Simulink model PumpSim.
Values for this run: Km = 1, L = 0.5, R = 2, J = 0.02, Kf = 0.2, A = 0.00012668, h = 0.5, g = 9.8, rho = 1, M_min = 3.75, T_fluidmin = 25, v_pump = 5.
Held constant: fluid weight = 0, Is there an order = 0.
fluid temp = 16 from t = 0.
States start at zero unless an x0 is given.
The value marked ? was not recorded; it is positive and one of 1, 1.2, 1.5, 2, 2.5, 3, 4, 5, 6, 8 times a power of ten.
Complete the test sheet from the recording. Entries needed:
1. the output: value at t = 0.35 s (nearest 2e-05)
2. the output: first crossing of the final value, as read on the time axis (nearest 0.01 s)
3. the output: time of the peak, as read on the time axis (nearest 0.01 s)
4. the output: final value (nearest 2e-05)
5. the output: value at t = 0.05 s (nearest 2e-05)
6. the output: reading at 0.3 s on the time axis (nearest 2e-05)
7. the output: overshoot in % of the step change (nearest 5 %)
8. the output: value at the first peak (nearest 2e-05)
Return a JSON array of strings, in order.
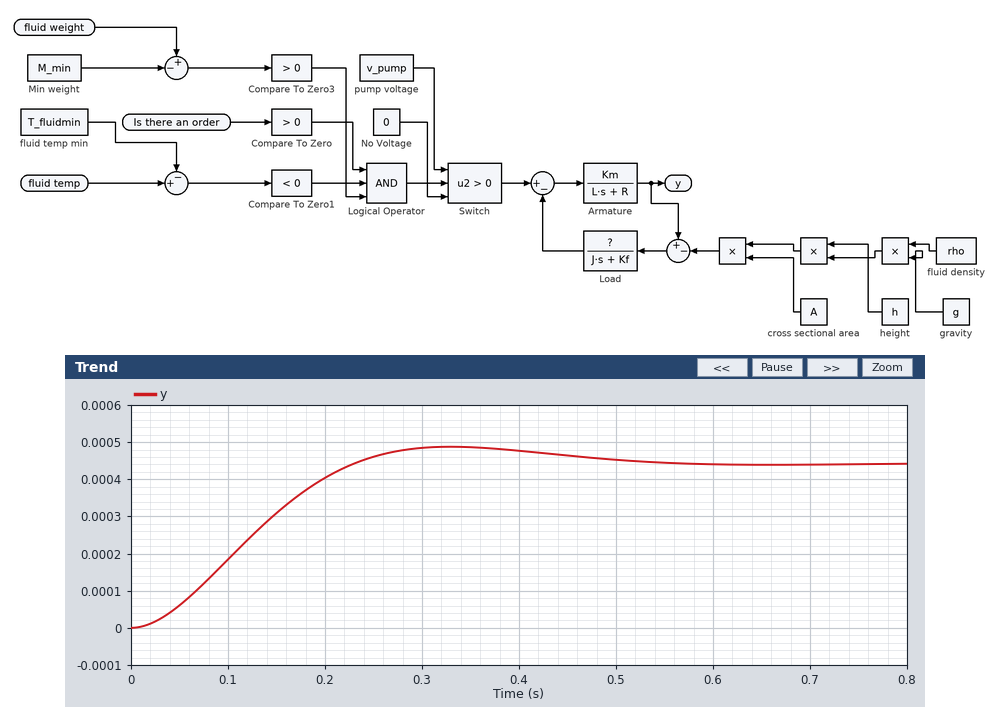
["0.00048", "0.23 s", "0.33 s", "0.00044", "0.00006", "0.00048", "10 %", "0.00048"]
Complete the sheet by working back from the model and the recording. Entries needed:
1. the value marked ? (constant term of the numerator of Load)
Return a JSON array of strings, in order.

["1"]
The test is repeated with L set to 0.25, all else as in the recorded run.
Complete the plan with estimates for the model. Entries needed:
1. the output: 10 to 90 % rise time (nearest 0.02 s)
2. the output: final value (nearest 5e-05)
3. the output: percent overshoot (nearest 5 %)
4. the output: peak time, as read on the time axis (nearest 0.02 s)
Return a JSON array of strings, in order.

["0.10 s", "0.00045", "15 %", "0.22 s"]
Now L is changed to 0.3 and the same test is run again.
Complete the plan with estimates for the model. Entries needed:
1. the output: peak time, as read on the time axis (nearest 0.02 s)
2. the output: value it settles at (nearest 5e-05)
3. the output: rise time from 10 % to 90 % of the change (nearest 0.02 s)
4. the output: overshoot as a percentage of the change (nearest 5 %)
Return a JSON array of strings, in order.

["0.24 s", "0.00045", "0.12 s", "15 %"]
